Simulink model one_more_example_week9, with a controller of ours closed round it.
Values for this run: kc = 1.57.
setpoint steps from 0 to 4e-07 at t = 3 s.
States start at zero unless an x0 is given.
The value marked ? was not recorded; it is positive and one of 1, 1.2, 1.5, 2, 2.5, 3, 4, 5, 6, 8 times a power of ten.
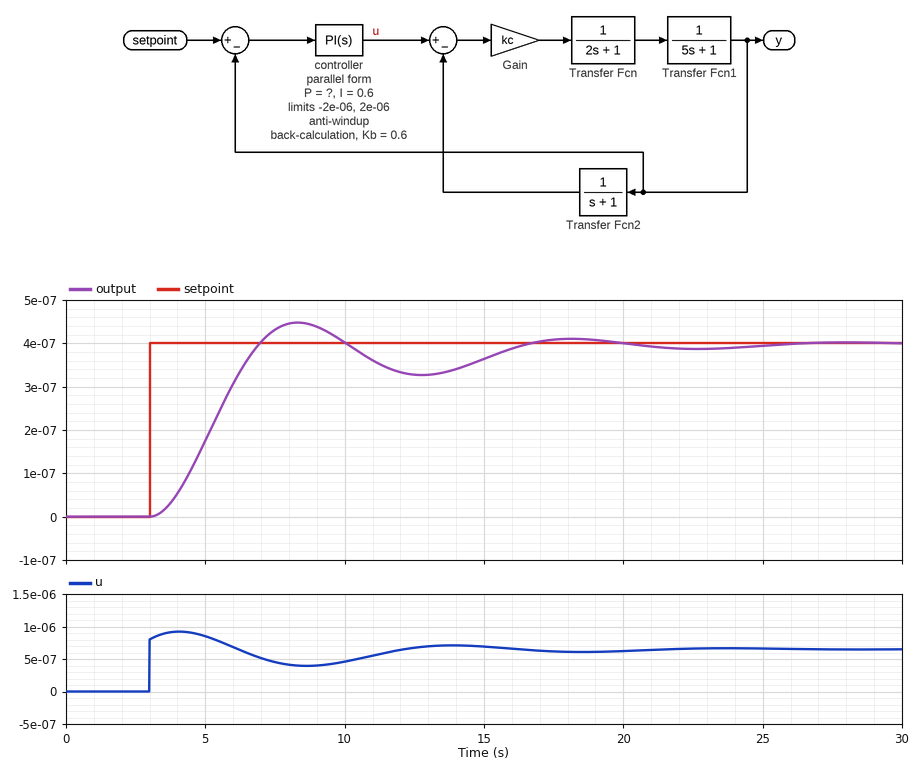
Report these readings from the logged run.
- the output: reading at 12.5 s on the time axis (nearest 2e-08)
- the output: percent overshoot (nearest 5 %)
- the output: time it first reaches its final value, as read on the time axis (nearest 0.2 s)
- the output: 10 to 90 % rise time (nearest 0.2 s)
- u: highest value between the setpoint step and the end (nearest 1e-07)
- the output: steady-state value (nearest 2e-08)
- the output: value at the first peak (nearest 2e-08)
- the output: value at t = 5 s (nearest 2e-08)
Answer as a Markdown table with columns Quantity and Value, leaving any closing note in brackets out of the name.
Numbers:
| Quantity | Value |
|---|---|
| the output: reading at 12.5 s on the time axis | 0.00000032 |
| the output: percent overshoot | 10 % |
| the output: time it first reaches its final value, as read on the time axis | 7.0 s |
| the output: 10 to 90 % rise time | 2.6 s |
| u: highest value between the setpoint step and the end | 0.0000009 |
| the output: steady-state value | 0.00000040 |
| the output: value at the first peak | 0.00000044 |
| the output: value at t = 5 s | 0.00000018 |
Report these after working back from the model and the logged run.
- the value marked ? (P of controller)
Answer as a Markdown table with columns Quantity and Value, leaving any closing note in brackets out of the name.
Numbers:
| Quantity | Value |
|---|---|
| the value marked ? | 2 |
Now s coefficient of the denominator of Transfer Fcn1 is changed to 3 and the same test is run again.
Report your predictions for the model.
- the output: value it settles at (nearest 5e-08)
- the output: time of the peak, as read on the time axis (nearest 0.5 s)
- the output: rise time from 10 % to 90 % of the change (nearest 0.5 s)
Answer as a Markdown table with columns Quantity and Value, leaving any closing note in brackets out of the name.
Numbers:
| Quantity | Value |
|---|---|
| the output: value it settles at | 0.00000040 |
| the output: time of the peak, as read on the time axis | 7.0 s |
| the output: rise time from 10 % to 90 % of the change | 2.0 s |
